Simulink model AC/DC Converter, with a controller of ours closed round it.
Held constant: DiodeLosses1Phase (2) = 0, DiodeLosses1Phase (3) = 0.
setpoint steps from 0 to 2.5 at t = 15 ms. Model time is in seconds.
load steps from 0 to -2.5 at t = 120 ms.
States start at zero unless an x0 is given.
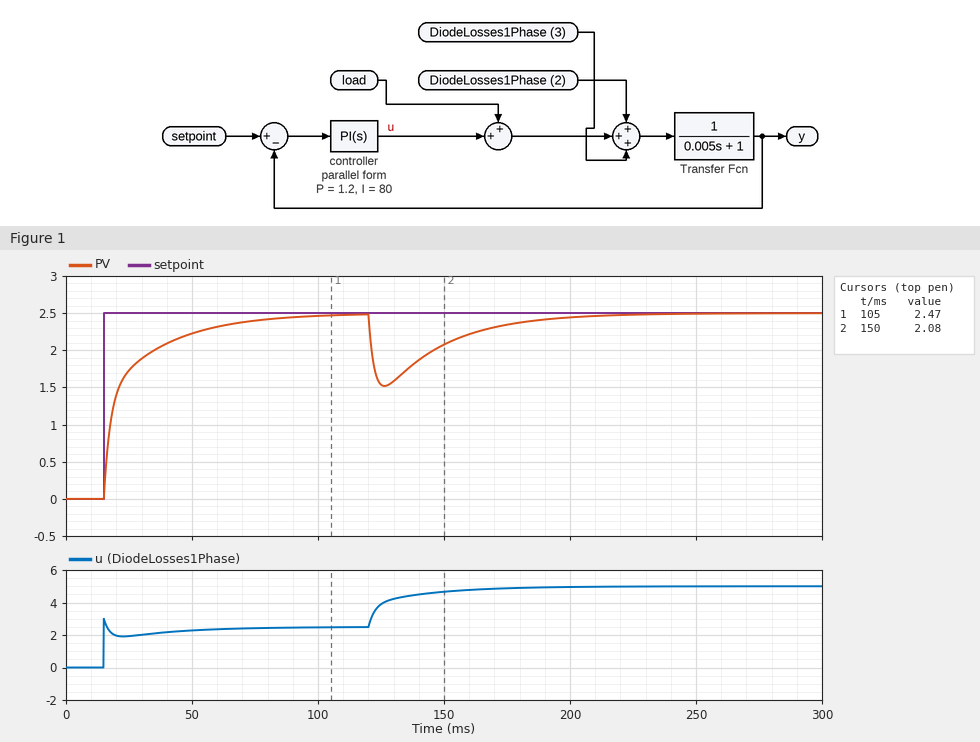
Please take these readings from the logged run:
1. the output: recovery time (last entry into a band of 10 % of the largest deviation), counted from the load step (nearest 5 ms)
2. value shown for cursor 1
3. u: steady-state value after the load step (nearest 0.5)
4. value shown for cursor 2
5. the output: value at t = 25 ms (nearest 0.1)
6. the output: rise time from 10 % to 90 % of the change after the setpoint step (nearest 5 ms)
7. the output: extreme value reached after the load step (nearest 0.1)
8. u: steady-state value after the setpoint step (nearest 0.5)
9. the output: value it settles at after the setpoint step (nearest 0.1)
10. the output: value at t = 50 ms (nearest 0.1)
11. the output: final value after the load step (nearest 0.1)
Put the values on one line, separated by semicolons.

65 ms; 2.47; 5.0; 2.08; 1.7; 35 ms; 1.5; 2.5; 2.5; 2.2; 2.5
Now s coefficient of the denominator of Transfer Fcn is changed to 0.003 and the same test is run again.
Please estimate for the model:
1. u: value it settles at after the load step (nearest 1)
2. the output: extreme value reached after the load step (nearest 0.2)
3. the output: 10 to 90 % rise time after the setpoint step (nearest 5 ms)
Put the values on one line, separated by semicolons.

5; 1.4; 40 ms
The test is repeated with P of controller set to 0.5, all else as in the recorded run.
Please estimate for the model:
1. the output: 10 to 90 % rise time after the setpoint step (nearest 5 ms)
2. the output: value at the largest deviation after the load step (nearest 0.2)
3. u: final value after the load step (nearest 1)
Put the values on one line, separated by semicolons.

30 ms; 1.2; 5
